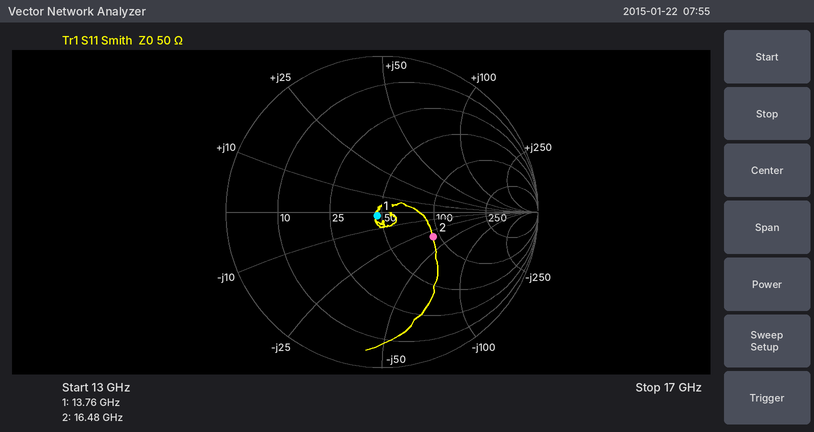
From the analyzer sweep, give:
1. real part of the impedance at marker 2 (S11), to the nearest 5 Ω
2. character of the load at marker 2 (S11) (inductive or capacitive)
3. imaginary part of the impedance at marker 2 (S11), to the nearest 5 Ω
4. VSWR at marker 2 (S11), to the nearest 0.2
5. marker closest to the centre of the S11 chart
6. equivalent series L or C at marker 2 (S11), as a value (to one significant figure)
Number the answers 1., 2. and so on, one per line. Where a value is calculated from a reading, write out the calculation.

1. 90 Ω
2. capacitive
3. -35 Ω
4. 2.2
5. marker 1
6. C = 1/(2π × 16.48 GHz × 35 Ω) ≈ 276 fF, so 300 fF to one significant figure
